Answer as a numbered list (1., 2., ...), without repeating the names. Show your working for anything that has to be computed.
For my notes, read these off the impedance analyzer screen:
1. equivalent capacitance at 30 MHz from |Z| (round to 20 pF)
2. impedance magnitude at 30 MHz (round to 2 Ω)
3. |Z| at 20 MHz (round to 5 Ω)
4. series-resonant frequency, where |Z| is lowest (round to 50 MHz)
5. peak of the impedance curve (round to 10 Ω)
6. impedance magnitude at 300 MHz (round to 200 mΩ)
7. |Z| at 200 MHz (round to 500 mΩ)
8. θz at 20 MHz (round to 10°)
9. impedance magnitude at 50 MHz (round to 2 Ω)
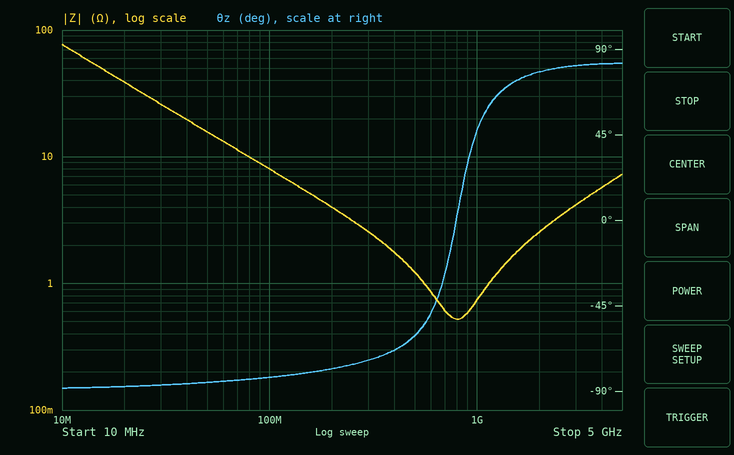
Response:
1. C = 1/(2π × 30 MHz × 26 Ω) ≈ 204 pF, so 200 pF to the nearest 20 pF
2. 26 Ω
3. 40 Ω
4. 800 MHz
5. 80 Ω
6. 2.6 Ω
7. 4.0 Ω
8. -90°
9. 16 Ω
